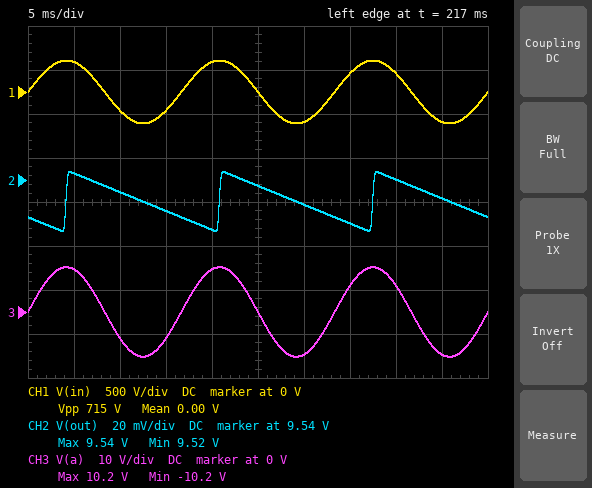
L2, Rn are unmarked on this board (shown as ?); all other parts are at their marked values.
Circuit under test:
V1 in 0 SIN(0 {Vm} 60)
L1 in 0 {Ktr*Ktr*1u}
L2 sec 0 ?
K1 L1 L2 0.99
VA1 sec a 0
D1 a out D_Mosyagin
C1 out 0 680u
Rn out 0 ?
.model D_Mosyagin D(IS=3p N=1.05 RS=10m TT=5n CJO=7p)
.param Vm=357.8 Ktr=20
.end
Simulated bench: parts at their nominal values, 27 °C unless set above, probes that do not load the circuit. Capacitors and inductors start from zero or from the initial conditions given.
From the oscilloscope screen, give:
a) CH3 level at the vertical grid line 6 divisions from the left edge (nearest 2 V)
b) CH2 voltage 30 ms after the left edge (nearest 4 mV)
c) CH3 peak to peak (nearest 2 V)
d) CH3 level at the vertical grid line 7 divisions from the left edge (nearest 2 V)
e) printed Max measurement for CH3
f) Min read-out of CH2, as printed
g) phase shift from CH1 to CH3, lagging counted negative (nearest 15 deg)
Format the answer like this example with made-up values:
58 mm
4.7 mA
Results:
-10 V
9.528 V
20 V
6 V
10.2 V
9.52 V
0 deg
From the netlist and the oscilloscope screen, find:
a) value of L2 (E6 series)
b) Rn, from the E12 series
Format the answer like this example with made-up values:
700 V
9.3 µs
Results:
330 nH
8.2 kΩ
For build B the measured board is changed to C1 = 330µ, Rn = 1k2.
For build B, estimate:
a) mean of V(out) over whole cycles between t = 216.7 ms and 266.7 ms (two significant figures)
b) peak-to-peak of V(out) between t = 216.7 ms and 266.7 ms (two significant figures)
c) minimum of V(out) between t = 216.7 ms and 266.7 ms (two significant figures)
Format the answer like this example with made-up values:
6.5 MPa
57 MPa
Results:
9.4 V
370 mV
9.2 V
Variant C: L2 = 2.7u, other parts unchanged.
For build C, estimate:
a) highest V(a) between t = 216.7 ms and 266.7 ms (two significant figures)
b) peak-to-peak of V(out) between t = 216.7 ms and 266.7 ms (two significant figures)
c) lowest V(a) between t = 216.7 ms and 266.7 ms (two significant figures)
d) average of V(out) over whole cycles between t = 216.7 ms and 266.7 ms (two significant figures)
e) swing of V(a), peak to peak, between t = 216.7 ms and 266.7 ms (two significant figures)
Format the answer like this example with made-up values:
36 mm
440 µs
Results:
29 V
82 mV
-29 V
28 V
58 V
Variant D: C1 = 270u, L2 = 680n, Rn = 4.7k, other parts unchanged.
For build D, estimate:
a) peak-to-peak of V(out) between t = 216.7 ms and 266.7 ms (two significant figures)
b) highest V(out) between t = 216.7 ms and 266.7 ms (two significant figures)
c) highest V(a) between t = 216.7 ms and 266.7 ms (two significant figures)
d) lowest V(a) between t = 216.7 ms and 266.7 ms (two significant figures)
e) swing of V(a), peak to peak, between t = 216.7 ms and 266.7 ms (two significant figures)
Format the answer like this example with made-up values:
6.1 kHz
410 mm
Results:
170 mV
14 V
15 V
-15 V
29 V
